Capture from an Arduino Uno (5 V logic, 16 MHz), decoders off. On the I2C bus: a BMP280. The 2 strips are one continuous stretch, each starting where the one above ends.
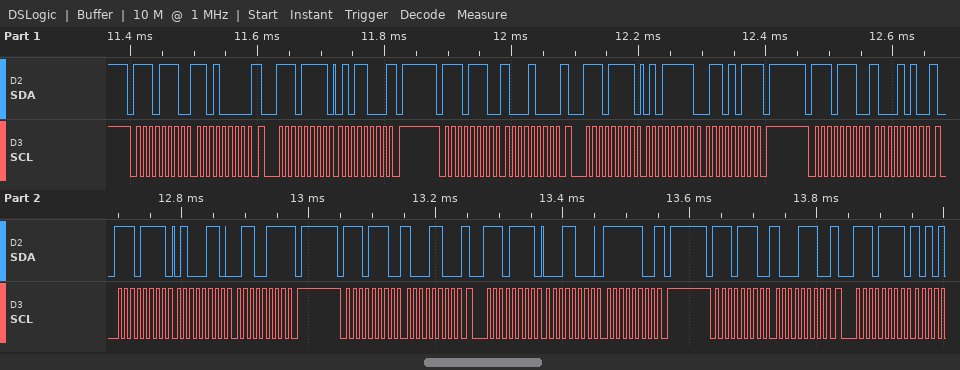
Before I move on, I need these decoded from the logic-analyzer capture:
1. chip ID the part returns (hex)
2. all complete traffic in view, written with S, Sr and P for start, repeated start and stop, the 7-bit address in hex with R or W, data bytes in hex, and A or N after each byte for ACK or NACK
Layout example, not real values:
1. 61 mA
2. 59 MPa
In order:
1. 0x58
2. S 77W A D0 A Sr 77R A 58 N P S 77W A 88 A Sr 77R A 5F A 6B N P S 77W A 8A A Sr 77R A 46 A 67 N P S 77W A 8C A Sr 77R A 18 A FC N P S 77W A 8E A Sr 77R A
